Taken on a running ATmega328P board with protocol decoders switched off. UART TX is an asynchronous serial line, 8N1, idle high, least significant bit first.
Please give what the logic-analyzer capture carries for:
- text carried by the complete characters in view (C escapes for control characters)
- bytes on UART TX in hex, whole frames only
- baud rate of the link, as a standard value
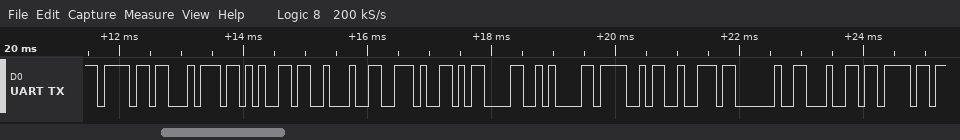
"ote\".\r\nOr do"
0x6F 0x74 0x65 0x22 0x2E 0x0D 0x0A 0x4F 0x72 0x20 0x64 0x6F
9600 baud
